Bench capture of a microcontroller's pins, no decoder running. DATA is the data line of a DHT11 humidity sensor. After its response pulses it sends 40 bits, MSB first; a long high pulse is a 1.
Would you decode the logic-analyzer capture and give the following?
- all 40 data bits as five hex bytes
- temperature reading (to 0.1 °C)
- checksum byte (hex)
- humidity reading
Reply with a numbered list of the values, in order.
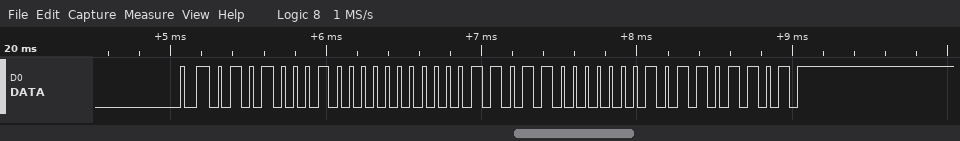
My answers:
1. 51 00 1B 01 6D
2. 27.1 °C
3. 0x6D
4. 81 %
